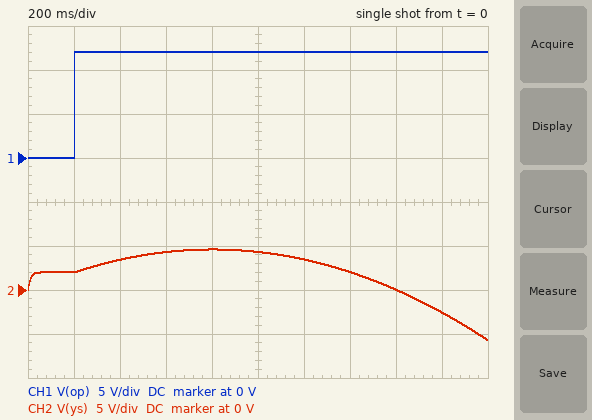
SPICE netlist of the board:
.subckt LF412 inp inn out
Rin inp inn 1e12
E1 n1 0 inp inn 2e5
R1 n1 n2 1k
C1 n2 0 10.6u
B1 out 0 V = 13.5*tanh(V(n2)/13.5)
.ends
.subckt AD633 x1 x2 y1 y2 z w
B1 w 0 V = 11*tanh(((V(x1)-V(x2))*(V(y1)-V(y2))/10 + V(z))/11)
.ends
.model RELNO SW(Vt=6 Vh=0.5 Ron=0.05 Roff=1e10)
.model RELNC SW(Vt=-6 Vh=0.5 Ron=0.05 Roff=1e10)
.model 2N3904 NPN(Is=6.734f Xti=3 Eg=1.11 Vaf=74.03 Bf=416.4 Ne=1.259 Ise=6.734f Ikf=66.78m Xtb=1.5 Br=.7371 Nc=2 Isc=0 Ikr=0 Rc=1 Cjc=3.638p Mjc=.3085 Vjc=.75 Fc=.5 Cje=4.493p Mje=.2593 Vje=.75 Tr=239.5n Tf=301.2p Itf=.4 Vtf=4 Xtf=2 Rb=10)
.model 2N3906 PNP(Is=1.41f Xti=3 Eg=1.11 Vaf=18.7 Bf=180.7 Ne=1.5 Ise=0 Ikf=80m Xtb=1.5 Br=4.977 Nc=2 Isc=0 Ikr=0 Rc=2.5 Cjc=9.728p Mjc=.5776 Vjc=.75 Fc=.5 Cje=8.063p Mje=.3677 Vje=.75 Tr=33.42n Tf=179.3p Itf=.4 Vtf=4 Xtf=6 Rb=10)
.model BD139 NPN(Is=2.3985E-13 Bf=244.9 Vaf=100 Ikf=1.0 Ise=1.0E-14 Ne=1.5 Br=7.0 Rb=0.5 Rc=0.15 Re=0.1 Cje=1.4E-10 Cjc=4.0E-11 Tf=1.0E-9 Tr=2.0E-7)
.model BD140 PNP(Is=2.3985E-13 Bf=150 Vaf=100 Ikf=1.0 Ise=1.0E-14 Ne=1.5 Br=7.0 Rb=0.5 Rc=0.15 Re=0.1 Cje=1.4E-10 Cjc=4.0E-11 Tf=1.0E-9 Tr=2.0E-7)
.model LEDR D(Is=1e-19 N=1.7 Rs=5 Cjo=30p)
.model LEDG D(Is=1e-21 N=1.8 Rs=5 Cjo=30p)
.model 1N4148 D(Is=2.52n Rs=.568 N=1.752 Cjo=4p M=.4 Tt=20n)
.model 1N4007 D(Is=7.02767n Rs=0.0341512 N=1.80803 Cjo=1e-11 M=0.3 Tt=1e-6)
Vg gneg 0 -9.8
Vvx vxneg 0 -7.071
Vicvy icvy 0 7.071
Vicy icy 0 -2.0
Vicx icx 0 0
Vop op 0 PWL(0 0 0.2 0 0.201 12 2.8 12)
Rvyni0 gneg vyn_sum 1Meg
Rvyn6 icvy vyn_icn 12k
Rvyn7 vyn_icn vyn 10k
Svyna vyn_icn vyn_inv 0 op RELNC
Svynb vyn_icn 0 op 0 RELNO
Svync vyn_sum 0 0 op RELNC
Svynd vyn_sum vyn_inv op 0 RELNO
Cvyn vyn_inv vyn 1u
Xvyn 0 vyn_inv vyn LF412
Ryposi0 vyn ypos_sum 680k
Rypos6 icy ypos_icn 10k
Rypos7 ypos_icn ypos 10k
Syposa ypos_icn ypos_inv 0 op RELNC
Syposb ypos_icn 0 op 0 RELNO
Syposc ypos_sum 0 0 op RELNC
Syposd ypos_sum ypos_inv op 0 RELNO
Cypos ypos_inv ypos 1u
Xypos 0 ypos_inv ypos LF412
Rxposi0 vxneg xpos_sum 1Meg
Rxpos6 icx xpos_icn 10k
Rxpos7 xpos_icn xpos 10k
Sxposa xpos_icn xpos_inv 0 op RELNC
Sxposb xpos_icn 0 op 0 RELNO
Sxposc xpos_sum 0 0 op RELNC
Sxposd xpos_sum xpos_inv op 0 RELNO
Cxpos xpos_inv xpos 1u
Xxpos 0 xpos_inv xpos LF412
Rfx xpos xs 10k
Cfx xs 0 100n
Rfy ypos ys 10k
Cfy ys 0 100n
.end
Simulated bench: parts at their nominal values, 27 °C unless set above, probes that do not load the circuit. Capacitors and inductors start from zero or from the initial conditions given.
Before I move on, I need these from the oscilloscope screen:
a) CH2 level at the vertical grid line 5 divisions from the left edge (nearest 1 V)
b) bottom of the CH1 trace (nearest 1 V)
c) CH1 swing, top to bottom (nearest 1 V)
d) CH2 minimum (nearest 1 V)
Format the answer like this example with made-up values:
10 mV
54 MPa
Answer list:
4 V
0 V
12 V
-6 V
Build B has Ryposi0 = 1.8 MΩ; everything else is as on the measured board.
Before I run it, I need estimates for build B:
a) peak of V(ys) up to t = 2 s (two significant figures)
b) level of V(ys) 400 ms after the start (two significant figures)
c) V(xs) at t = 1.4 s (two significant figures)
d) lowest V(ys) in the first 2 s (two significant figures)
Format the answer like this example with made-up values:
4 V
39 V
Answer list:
3.0 V
2.5 V
8.5 V
-920 mV
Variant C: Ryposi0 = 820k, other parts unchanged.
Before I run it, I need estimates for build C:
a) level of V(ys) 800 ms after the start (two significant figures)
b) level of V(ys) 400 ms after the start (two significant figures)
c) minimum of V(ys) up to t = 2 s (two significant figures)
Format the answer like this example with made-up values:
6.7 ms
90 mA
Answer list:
4.2 V
3.2 V
-4.4 V
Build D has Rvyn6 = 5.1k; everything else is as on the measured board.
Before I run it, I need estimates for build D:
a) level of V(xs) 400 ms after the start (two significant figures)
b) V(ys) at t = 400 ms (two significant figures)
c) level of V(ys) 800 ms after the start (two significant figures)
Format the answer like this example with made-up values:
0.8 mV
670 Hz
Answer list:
1.4 V
5.7 V
11 V
